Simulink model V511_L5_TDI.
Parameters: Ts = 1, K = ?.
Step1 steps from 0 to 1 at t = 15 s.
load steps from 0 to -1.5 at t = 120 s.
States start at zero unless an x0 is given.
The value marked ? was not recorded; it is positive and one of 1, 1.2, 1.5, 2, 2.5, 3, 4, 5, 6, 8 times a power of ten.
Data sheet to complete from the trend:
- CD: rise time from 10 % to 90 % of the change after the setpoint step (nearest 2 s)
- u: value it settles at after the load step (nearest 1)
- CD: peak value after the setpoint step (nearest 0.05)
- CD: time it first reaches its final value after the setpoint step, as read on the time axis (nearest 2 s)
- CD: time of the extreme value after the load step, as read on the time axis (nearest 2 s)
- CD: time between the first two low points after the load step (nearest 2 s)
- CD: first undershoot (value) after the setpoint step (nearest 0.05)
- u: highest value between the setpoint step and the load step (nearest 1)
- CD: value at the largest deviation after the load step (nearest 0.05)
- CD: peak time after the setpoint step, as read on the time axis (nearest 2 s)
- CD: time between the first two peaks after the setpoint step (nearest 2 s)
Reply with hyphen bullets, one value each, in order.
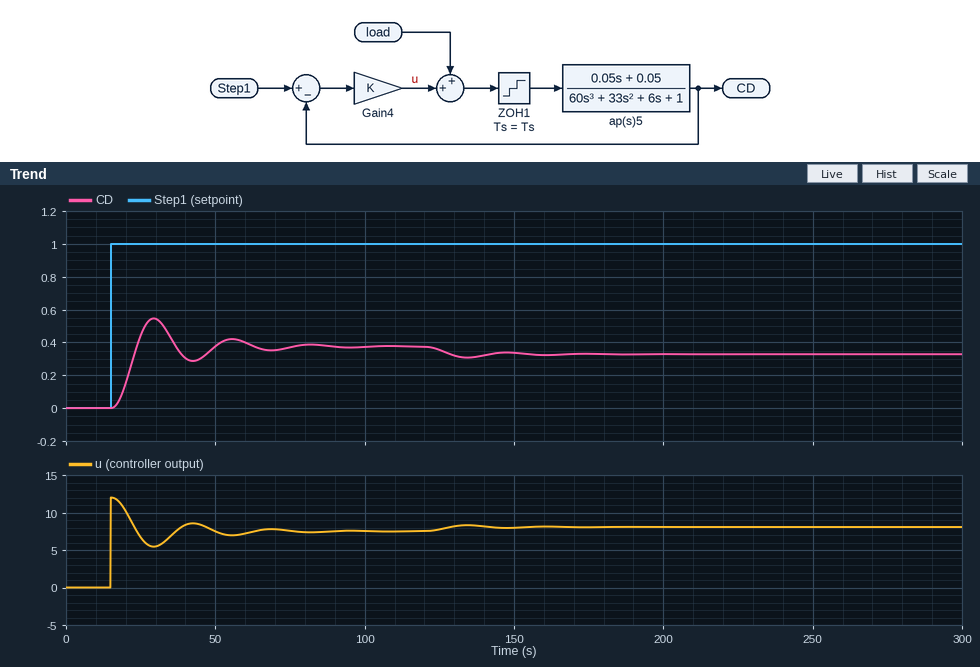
- 6 s
- 8
- 0.55
- 24 s
- 134 s
- 26 s
- 0.30
- 12
- 0.30
- 30 s
- 26 s
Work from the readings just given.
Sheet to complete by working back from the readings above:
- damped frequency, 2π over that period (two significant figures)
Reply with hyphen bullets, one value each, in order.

- 0.24 rad/s
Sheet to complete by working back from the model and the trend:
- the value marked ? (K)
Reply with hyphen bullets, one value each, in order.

- 12
